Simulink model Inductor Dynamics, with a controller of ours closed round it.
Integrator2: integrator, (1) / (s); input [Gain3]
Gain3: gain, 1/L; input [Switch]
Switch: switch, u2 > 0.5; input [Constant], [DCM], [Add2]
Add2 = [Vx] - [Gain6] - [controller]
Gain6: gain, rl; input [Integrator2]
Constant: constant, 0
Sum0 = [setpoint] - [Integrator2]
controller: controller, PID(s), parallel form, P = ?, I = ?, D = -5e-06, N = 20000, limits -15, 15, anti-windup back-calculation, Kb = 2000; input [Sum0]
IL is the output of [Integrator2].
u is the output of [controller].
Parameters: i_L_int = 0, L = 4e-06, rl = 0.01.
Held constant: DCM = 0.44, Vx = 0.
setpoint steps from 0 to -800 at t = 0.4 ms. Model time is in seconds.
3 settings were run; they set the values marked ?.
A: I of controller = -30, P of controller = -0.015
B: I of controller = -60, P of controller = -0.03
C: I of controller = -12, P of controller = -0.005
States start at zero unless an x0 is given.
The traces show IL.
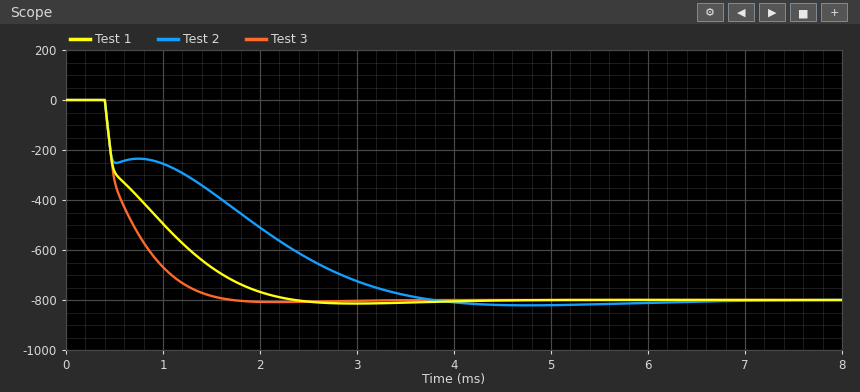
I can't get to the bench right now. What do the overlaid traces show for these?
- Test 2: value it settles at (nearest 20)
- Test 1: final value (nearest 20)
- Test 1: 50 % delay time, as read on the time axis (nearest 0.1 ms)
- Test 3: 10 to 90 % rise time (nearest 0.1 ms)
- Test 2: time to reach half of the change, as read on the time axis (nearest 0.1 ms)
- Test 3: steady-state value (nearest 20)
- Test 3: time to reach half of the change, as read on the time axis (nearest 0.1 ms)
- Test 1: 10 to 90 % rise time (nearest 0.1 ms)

-800
-800
0.8 ms
0.7 ms
1.6 ms
-800
0.6 ms
1.3 ms
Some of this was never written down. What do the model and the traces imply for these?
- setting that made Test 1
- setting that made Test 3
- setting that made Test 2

A
B
C
